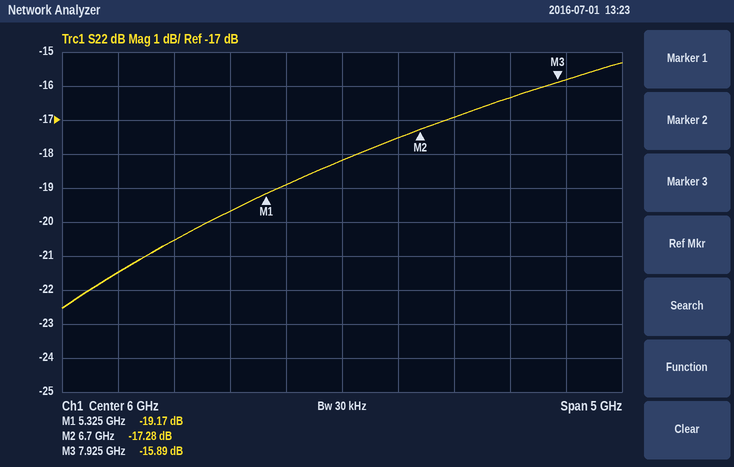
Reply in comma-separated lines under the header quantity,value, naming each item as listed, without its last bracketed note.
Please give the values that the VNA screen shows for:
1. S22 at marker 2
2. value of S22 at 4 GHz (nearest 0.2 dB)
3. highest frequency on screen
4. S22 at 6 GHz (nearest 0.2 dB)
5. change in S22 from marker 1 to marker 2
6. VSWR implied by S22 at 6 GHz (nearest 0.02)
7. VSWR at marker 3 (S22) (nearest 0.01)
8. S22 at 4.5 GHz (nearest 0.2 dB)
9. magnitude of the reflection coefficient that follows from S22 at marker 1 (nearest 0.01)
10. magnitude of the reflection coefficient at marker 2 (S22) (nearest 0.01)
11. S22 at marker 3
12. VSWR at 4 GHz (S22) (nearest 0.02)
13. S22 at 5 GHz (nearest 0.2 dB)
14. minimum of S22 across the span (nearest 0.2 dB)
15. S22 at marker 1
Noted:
quantity,value
S22 at marker 2,-17.28 dB
value of S22 at 4 GHz,-21.4 dB
highest frequency on screen,8.5 GHz
S22 at 6 GHz,-18.2 dB
change in S22 from marker 1 to marker 2,1.89 dB
VSWR implied by S22 at 6 GHz,1.28
VSWR at marker 3 (S22),1.38
S22 at 4.5 GHz,-20.6 dB
magnitude of the reflection coefficient that follows from S22 at marker 1,0.11
magnitude of the reflection coefficient at marker 2 (S22),0.14
S22 at marker 3,-15.89 dB
VSWR at 4 GHz (S22),1.18
S22 at 5 GHz,-19.6 dB
minimum of S22 across the span,-22.6 dB
S22 at marker 1,-19.17 dB
